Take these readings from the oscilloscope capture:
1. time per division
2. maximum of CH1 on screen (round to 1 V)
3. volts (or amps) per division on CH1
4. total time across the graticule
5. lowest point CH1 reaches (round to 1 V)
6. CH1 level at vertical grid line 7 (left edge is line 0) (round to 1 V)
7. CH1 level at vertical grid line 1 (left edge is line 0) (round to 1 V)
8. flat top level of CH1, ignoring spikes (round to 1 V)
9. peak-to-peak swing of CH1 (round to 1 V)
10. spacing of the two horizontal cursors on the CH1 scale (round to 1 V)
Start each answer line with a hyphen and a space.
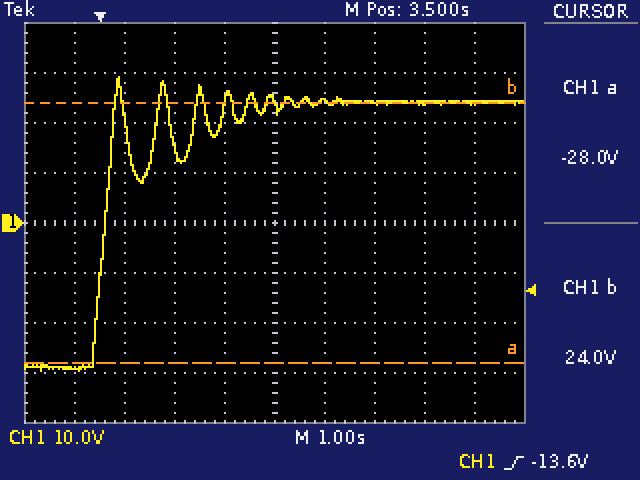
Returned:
- 1 s
- 29 V
- 10 V
- 10 s
- -30 V
- 24 V
- -29 V
- 24 V
- 59 V
- 52 V
